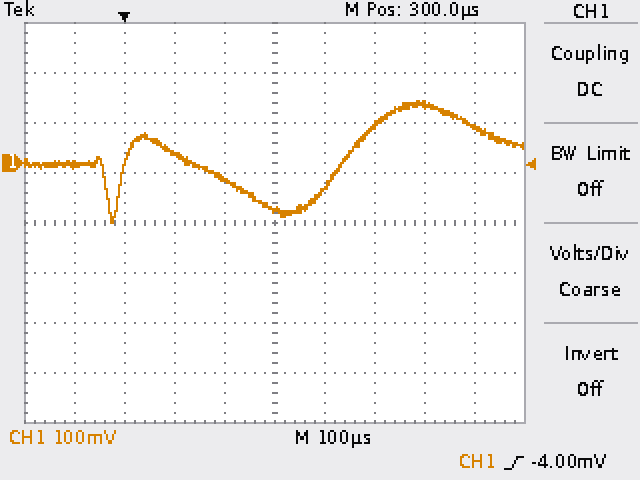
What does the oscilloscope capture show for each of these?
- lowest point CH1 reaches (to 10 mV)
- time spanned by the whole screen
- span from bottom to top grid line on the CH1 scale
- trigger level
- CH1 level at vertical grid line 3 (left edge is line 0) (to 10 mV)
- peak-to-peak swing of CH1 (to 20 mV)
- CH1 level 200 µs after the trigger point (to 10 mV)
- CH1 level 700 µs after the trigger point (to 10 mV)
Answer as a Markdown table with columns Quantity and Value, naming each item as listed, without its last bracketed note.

| Quantity | Value |
|---|---|
| lowest point CH1 reaches | -120 mV |
| time spanned by the whole screen | 1 ms |
| span from bottom to top grid line on the CH1 scale | 800 mV |
| trigger level | -4.00 mV |
| CH1 level at vertical grid line 3 (left edge is line 0) | 20 mV |
| peak-to-peak swing of CH1 | 240 mV |
| CH1 level 200 µs after the trigger point | -30 mV |
| CH1 level 700 µs after the trigger point | 70 mV |
